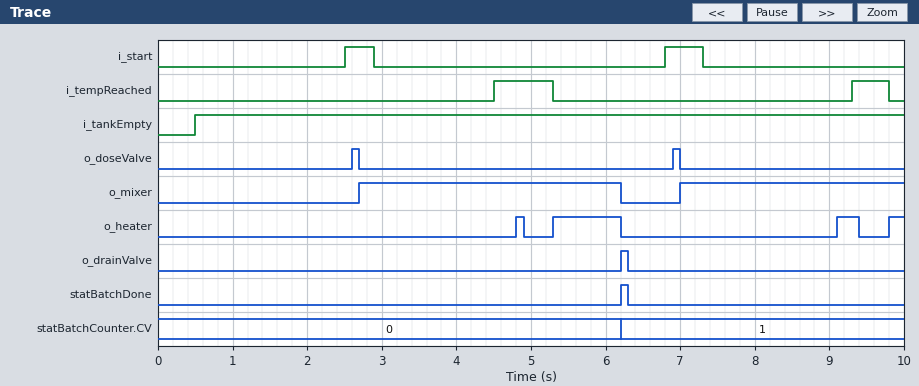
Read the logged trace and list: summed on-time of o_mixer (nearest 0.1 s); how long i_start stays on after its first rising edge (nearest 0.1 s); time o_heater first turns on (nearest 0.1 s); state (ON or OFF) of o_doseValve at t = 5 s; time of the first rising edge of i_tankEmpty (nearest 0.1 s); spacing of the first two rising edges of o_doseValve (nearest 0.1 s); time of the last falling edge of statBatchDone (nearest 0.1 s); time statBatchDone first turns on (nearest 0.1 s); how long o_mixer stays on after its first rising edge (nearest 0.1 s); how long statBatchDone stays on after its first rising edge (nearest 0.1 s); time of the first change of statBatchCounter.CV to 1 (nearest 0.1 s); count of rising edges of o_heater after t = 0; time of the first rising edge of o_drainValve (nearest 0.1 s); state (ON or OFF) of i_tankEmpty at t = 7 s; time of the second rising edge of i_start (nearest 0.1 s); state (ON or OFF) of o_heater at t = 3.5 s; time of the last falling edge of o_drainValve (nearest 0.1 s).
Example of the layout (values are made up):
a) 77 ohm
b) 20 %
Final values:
a) 6.5 s
b) 0.4 s
c) 4.8 s
d) OFF
e) 0.5 s
f) 4.3 s
g) 6.3 s
h) 6.2 s
i) 3.5 s
j) 0.1 s
k) 6.2 s
l) 4
m) 6.2 s
n) ON
o) 6.8 s
p) OFF
q) 6.3 s
